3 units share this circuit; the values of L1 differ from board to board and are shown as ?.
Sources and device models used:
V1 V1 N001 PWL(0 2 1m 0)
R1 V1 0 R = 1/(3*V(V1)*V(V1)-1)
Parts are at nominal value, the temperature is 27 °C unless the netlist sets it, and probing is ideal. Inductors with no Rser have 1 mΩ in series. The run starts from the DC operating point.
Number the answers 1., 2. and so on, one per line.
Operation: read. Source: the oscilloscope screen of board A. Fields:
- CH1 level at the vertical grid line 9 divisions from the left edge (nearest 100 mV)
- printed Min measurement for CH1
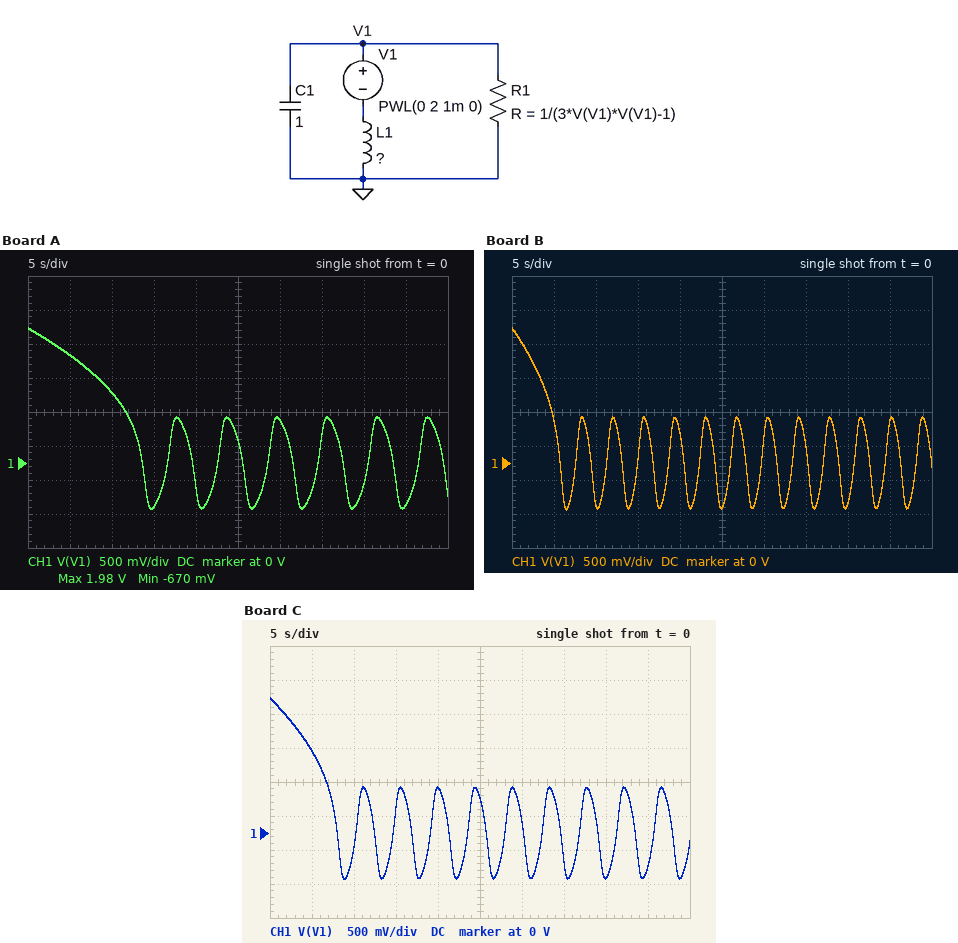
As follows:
1. -600 mV
2. -670 mV
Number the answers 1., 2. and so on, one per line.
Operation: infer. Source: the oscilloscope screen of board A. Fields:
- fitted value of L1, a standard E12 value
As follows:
1. 820 mH
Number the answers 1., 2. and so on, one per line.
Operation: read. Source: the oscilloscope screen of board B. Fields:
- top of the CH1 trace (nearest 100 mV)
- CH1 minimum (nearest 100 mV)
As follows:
1. 2.0 V
2. -700 mV
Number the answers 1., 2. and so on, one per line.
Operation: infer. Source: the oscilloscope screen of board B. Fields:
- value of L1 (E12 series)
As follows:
1. 330 mH
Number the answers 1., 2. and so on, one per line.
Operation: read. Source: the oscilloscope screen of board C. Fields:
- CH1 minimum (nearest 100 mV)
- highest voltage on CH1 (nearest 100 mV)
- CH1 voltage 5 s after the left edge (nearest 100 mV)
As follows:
1. -700 mV
2. 2.0 V
3. 1.2 V
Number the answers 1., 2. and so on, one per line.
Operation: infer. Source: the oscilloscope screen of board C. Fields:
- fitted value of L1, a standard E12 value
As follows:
1. 470 mH
